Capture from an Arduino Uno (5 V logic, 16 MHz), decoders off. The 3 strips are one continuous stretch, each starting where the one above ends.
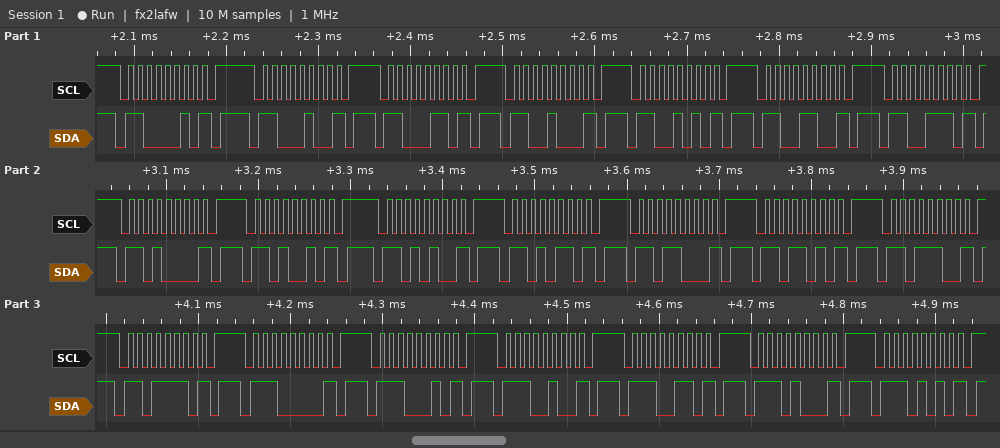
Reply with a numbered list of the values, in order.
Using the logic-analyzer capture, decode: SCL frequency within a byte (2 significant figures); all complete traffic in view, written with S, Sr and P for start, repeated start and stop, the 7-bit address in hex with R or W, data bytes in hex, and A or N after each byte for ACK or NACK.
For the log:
1. 100 kHz
2. S 61W N P S 62W N P S 63W N P S 64W N P S 65W N P S 66W N P S 67W N P S 68W N P S 69W N P S 6AW N P S 6BW N P S 6CW N P S 6DW N P S 6EW N P S 6FW N P S 70W N P S 71W N P S 72W N P S 73W N P S 74W N P S 75W N P
